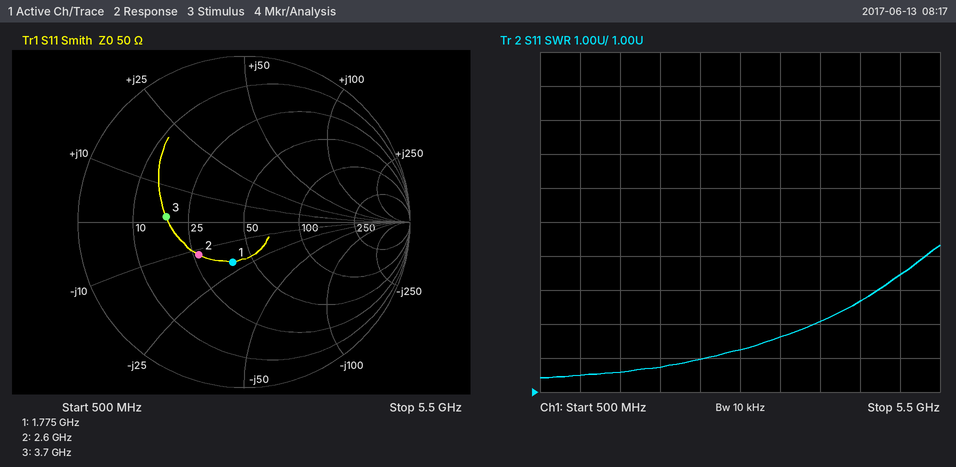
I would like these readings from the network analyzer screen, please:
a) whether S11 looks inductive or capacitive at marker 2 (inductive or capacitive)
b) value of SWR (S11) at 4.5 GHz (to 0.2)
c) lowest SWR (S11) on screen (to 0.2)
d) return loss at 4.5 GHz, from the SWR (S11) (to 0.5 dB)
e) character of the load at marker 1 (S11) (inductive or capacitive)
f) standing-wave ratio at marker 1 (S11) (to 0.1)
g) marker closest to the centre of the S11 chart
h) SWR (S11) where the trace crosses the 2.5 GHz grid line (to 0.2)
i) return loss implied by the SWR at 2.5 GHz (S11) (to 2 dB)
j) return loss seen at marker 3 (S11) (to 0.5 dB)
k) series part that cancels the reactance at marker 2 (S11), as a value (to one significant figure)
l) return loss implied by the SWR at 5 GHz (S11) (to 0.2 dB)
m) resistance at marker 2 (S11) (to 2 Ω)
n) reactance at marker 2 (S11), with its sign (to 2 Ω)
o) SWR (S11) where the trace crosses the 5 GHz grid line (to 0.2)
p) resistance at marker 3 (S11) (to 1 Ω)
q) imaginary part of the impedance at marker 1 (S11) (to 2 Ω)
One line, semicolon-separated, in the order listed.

capacitive; 3.6; 1.4; 5.0 dB; capacitive; 1.7; marker 1; 2.0; 10 dB; 6.5 dB; 700 pH; 4.0 dB; 26 Ω; -12 Ω; 4.4; 18 Ω; -20 Ω
